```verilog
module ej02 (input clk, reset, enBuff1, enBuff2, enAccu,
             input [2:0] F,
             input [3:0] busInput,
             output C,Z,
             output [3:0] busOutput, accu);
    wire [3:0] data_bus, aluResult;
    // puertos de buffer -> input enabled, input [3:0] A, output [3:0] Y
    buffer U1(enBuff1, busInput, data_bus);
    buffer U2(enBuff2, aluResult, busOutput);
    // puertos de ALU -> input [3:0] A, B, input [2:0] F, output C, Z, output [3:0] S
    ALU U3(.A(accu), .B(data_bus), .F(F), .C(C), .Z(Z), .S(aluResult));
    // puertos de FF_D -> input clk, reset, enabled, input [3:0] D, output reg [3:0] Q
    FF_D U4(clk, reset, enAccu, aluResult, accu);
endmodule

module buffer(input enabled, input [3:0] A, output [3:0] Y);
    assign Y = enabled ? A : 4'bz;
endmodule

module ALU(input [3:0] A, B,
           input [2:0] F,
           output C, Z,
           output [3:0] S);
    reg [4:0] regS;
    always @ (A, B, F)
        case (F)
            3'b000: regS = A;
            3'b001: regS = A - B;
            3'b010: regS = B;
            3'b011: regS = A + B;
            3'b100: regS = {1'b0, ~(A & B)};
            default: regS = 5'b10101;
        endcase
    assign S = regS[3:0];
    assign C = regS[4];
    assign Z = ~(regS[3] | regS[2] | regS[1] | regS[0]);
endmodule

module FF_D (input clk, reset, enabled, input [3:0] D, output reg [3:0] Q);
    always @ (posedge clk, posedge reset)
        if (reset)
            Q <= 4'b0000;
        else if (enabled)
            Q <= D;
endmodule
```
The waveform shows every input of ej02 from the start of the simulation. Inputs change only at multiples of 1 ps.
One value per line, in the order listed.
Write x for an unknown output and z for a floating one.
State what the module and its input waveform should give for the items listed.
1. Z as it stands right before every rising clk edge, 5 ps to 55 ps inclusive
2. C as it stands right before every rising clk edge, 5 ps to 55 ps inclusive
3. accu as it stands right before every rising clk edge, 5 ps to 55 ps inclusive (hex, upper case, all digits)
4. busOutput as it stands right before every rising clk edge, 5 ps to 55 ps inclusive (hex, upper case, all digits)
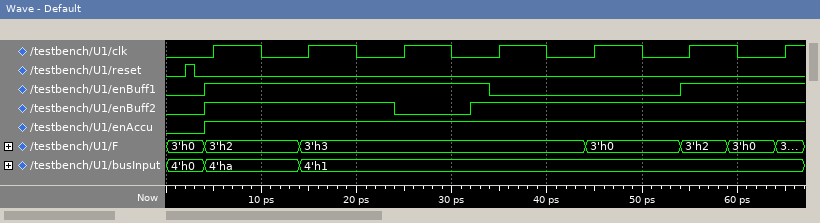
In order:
0 0 0 x x 0
0 0 0 x 0 0
0, A, B, C, x, x
A, B, z, x, x, 1
